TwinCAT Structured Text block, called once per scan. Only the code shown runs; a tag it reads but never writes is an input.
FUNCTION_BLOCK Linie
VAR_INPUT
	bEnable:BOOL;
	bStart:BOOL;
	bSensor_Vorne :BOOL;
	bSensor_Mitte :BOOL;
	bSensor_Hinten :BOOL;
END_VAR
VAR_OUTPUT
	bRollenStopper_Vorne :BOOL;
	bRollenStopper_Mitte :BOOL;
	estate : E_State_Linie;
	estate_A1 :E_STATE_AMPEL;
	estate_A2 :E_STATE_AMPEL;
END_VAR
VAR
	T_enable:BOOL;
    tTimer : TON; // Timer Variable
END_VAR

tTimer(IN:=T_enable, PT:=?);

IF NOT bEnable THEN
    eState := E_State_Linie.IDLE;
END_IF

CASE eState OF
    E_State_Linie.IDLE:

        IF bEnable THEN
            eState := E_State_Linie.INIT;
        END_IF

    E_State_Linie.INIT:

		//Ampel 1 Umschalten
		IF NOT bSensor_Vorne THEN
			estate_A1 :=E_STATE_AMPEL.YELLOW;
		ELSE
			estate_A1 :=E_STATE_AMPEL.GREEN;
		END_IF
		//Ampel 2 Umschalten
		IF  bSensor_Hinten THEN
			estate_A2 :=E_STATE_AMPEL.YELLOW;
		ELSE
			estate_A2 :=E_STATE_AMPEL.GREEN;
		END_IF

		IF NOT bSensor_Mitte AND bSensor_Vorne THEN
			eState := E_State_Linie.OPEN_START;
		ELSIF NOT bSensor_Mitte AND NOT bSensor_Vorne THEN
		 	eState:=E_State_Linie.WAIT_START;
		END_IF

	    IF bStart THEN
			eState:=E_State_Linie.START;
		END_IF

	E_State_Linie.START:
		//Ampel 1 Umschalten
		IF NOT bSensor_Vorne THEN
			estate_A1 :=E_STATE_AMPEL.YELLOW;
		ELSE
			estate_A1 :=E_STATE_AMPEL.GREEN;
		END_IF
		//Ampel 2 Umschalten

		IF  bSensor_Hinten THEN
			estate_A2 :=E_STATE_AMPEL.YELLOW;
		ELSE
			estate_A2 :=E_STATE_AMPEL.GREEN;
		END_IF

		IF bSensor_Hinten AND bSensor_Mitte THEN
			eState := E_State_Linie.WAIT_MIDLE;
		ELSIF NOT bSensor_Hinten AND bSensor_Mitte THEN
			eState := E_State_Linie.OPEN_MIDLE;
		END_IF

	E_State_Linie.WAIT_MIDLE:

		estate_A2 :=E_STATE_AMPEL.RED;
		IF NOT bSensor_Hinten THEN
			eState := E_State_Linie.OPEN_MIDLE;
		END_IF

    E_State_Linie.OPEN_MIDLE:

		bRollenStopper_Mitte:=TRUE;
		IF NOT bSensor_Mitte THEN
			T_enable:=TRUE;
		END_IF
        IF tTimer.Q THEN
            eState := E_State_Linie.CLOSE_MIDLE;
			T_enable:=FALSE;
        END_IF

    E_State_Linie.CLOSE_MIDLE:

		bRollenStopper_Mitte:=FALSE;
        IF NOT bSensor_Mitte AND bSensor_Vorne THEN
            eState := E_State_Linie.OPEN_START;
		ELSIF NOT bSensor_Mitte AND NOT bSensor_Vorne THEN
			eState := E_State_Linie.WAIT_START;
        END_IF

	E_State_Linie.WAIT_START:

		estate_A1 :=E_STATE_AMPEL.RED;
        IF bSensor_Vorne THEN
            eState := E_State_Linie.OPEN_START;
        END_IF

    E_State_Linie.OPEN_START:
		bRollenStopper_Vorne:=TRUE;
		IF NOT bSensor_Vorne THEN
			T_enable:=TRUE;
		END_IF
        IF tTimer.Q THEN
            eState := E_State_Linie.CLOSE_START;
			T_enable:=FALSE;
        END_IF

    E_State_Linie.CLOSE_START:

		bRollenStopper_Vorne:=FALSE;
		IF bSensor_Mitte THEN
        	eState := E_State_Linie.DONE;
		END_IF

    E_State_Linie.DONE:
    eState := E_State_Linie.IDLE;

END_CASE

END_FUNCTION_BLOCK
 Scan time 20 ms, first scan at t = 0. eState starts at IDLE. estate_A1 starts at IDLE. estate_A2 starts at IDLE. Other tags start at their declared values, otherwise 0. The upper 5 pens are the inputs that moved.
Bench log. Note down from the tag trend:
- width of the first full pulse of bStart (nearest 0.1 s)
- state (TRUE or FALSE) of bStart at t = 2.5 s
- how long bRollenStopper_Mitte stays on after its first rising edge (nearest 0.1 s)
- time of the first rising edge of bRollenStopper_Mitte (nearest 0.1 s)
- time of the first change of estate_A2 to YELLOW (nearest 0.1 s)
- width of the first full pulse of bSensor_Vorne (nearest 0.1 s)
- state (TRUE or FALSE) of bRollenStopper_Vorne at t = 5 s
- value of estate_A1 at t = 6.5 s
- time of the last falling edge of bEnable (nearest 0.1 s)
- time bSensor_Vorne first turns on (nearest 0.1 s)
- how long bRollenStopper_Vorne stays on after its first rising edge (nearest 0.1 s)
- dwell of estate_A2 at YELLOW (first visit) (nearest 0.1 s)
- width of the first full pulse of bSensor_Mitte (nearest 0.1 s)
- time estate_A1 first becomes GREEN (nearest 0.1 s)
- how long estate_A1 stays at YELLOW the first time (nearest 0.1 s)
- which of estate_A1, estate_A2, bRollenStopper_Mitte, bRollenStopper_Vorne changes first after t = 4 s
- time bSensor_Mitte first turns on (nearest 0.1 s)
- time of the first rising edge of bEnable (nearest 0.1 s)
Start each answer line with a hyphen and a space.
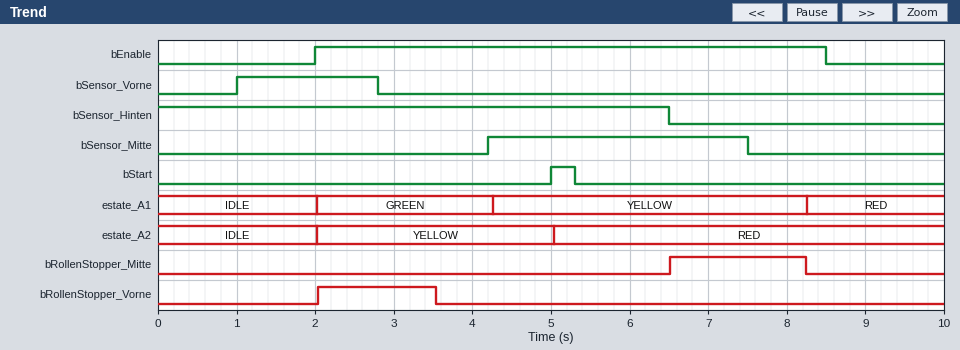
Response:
- 0.3 s
- FALSE
- 1.7 s
- 6.5 s
- 2.0 s
- 1.8 s
- FALSE
- YELLOW
- 8.5 s
- 1.0 s
- 1.5 s
- 3.0 s
- 3.3 s
- 2.0 s
- 4.0 s
- estate_A1
- 4.2 s
- 2.0 s
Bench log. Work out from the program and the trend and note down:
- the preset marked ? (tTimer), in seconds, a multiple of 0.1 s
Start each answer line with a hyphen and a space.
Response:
- 0.7 s
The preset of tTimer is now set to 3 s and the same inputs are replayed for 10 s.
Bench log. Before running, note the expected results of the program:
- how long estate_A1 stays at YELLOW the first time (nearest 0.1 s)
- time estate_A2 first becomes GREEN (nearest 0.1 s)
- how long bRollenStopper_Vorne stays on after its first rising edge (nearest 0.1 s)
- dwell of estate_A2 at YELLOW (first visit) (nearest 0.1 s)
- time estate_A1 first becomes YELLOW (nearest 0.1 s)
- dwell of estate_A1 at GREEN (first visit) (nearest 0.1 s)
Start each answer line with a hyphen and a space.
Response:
- 1.6 s
- 6.5 s
- 3.8 s
- 4.5 s
- 5.9 s
- 3.9 s
